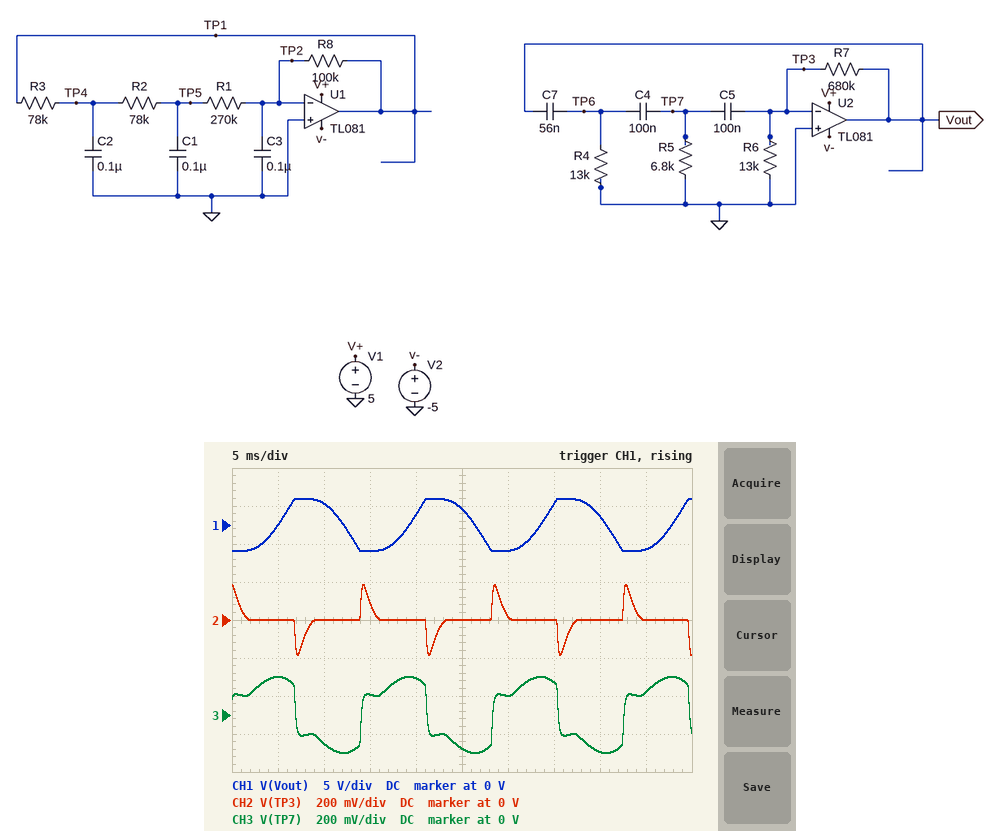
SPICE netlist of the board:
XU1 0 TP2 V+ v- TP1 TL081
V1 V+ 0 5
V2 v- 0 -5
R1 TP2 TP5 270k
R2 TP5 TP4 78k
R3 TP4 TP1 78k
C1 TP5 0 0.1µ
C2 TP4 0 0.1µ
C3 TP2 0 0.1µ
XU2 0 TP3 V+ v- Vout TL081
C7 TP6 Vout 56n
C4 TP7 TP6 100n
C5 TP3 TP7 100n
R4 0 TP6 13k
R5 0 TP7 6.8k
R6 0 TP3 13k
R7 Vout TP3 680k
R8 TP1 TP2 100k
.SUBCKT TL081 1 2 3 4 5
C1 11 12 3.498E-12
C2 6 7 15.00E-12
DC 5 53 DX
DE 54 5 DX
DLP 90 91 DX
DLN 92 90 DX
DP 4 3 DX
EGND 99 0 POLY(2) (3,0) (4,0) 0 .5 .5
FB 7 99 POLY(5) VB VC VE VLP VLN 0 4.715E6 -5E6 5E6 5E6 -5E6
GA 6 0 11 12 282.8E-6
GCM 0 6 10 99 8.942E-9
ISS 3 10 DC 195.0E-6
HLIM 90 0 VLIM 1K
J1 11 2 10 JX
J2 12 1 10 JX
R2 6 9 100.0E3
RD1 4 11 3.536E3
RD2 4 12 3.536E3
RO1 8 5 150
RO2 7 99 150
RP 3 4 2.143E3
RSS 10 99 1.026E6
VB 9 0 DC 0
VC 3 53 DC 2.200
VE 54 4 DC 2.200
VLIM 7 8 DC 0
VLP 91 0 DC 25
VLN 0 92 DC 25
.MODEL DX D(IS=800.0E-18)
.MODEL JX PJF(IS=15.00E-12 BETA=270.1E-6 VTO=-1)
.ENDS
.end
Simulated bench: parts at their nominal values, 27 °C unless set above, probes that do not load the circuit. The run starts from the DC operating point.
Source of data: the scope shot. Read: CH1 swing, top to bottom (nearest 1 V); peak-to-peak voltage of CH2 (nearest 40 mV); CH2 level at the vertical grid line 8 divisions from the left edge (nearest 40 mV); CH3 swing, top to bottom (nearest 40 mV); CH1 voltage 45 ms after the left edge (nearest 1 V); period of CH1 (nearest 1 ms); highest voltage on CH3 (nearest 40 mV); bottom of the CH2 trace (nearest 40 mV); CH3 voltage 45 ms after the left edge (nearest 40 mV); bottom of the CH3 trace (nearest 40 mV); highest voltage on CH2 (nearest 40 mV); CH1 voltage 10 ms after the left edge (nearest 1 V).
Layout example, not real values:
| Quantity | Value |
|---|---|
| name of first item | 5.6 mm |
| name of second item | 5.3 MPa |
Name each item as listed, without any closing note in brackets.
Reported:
| Quantity | Value |
|---|---|
| CH1 swing, top to bottom | 7 V |
| peak-to-peak voltage of CH2 | 360 mV |
| CH2 level at the vertical grid line 8 divisions from the left edge | 0 V |
| CH3 swing, top to bottom | 400 mV |
| CH1 voltage 45 ms after the left edge | -3 V |
| period of CH1 | 14 ms |
| highest voltage on CH3 | 200 mV |
| bottom of the CH2 trace | -200 mV |
| CH3 voltage 45 ms after the left edge | 120 mV |
| bottom of the CH3 trace | -200 mV |
| highest voltage on CH2 | 200 mV |
| CH1 voltage 10 ms after the left edge | 3 V |
